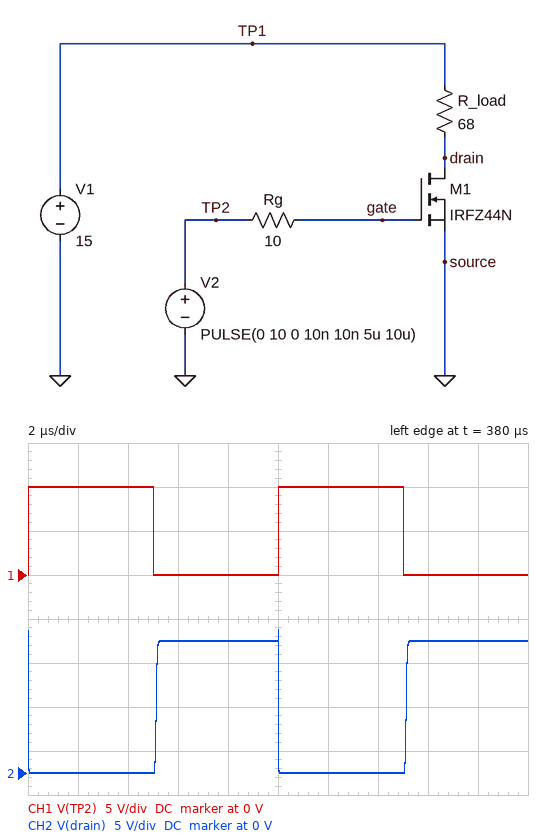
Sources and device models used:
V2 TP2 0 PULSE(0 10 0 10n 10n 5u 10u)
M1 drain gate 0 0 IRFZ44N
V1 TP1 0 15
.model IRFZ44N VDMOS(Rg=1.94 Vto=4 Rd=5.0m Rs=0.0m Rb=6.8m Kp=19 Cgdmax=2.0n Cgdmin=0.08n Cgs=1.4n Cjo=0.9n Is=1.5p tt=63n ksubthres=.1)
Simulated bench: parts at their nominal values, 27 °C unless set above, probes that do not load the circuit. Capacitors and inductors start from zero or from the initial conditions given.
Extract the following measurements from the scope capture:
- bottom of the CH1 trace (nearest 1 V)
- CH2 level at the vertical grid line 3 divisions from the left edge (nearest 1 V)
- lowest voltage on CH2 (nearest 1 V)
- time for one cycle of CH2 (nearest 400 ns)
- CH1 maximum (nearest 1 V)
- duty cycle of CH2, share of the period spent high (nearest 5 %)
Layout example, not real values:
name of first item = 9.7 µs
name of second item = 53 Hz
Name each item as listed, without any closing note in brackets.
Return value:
bottom of the CH1 trace = 0 V
CH2 level at the vertical grid line 3 divisions from the left edge = 15 V
lowest voltage on CH2 = 0 V
time for one cycle of CH2 = 10.0 µs
CH1 maximum = 10 V
duty cycle of CH2, share of the period spent high = 50 %
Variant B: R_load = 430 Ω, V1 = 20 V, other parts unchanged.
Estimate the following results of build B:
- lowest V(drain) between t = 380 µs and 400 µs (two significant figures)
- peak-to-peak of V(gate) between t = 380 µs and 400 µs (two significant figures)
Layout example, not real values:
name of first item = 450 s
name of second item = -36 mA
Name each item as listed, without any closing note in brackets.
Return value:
lowest V(drain) between t = 380 µs and 400 µs = -600 mV
peak-to-peak of V(gate) between t = 380 µs and 400 µs = 10 V
